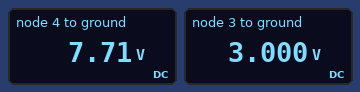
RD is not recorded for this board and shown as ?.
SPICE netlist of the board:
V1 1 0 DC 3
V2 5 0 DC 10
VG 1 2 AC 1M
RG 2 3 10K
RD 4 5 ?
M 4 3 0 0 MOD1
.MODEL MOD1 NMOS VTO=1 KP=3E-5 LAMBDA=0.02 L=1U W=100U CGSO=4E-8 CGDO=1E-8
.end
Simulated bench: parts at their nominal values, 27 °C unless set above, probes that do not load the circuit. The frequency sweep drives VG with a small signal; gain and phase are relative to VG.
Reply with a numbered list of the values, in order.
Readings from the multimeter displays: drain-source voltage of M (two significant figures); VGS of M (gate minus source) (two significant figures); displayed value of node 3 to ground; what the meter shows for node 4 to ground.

1. 7.7 V
2. 3.0 V
3. 3.000 V
4. 7.71 V
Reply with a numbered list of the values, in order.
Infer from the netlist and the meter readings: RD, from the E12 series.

1. 330 Ω
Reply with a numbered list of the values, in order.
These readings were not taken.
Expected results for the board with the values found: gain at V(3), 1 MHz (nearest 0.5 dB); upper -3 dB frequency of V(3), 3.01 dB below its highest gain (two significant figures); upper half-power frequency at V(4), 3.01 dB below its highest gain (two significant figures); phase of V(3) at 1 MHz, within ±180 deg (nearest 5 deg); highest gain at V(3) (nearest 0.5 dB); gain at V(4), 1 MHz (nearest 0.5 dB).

1. -1.0 dB
2. 2.2 MHz
3. 2.2 MHz
4. 155 deg
5. 0 dB
6. 6.0 dB
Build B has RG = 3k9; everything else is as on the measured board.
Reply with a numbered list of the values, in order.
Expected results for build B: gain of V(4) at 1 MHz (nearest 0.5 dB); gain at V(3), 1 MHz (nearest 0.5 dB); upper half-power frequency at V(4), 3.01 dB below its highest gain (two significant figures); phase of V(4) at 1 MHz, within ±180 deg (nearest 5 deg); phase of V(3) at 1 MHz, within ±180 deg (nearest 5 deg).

1. 6.5 dB
2. 0 dB
3. 5.6 MHz
4. -10 deg
5. 170 deg
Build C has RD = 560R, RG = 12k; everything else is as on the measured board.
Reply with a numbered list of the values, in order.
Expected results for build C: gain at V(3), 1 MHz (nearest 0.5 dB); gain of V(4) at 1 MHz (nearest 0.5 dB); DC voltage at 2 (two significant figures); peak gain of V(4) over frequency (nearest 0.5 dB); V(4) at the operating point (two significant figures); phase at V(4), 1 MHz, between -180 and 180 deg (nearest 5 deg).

1. -1.5 dB
2. 9.5 dB
3. 3.0 V
4. 11.0 dB
5. 6.2 V
6. -35 deg
